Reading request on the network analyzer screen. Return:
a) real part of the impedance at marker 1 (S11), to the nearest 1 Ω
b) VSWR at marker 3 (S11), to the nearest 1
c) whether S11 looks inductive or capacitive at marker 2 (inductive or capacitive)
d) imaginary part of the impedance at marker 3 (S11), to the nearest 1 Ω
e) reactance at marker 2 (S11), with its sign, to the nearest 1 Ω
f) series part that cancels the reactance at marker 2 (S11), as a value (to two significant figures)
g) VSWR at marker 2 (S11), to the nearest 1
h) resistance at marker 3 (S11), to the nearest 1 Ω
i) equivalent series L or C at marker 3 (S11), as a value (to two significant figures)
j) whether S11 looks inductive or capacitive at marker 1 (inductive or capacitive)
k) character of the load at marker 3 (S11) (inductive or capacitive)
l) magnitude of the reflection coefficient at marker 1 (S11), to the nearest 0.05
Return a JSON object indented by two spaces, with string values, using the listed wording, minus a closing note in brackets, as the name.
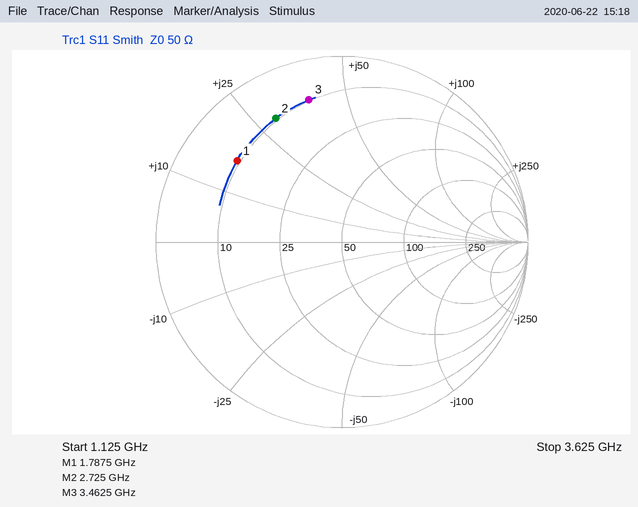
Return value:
{
  "real part of the impedance at marker 1 (S11), to the nearest 1 Ω": "9 Ω",
  "VSWR at marker 3 (S11), to the nearest 1": "8",
  "whether S11 looks inductive or capacitive at marker 2": "inductive",
  "imaginary part of the impedance at marker 3 (S11), to the nearest 1 Ω": "+39 Ω",
  "reactance at marker 2 (S11), with its sign, to the nearest 1 Ω": "+29 Ω",
  "series part that cancels the reactance at marker 2 (S11), as a value": "2.0 pF",
  "VSWR at marker 2 (S11), to the nearest 1": "7",
  "resistance at marker 3 (S11), to the nearest 1 Ω": "10 Ω",
  "equivalent series L or C at marker 3 (S11), as a value": "1.8 nH",
  "whether S11 looks inductive or capacitive at marker 1": "inductive",
  "character of the load at marker 3 (S11)": "inductive",
  "magnitude of the reflection coefficient at marker 1 (S11), to the nearest 0.05": "0.70"
}
